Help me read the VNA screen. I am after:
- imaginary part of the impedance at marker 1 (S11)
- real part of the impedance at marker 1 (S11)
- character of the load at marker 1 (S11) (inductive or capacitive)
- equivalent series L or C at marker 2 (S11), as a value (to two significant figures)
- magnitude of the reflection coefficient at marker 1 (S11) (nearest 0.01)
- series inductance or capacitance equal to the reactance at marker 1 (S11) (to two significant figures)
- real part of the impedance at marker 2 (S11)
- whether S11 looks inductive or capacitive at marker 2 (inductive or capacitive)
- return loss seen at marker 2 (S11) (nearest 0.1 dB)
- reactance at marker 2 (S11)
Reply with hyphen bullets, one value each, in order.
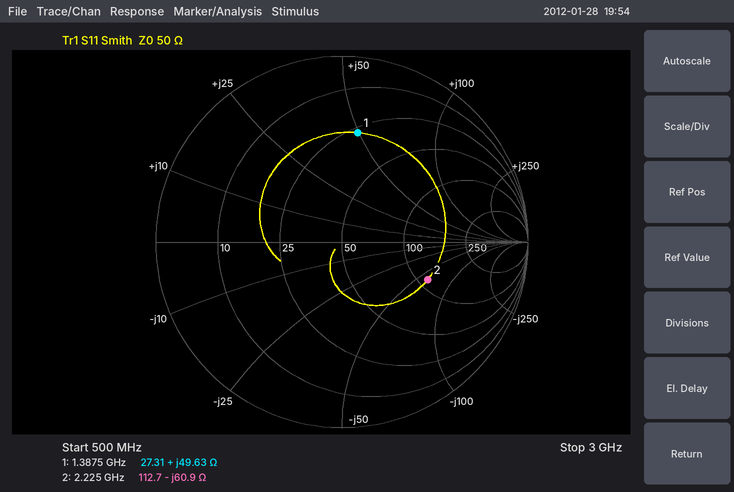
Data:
- +49.63 Ω
- 27.31 Ω
- inductive
- 1.2 pF
- 0.59
- 5.7 nH
- 112.7 Ω
- capacitive
- 6.0 dB
- -60.9 Ω
